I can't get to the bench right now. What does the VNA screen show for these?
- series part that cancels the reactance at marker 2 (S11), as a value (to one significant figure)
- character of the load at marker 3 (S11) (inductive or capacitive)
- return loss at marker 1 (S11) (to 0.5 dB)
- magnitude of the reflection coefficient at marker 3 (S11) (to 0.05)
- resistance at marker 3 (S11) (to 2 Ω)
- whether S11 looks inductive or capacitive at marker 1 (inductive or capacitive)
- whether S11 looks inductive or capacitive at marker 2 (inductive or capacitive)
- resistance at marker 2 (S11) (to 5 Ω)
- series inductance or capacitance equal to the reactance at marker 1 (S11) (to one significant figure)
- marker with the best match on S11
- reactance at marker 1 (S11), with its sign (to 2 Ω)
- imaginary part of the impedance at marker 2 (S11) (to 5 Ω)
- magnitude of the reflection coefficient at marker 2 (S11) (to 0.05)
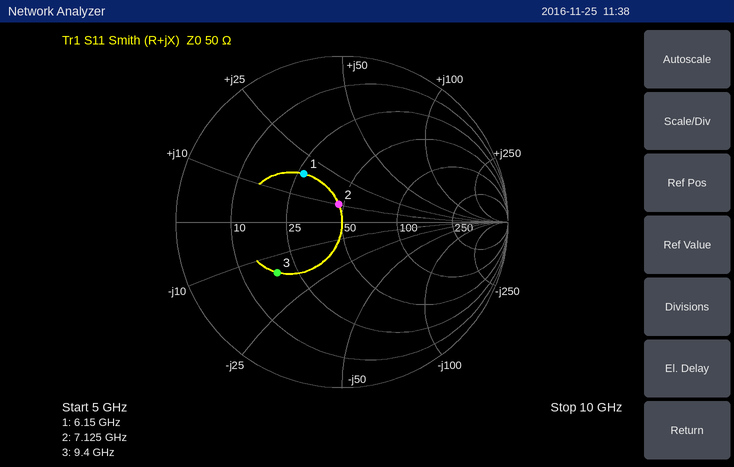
2 pF
capacitive
8.5 dB
0.50
18 Ω
inductive
inductive
45 Ω
500 pH
marker 2
+18 Ω
+10 Ω
0.10
